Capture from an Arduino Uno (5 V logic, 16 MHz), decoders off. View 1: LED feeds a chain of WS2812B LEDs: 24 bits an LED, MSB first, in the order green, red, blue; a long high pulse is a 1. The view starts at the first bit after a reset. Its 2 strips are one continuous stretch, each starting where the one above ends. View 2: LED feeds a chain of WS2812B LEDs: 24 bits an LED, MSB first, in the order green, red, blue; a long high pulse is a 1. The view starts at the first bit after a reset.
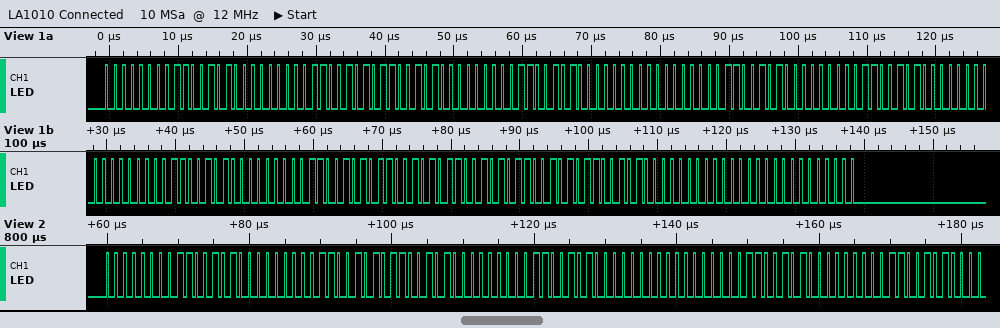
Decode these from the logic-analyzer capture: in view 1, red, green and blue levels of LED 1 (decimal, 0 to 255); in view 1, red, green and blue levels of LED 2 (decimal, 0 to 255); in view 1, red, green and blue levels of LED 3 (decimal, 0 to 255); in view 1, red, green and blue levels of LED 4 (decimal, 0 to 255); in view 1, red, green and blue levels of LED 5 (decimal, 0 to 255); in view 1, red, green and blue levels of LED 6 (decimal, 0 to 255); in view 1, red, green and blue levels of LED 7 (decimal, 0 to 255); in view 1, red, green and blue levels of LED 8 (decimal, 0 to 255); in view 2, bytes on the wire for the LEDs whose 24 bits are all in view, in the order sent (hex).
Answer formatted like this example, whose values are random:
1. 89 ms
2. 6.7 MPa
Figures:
1. 202, 0, 0
2. 202, 202, 0
3. 0, 202, 0
4. 0, 202, 202
5. 0, 0, 202
6. 202, 0, 202
7. 202, 202, 202
8. 0, 0, 0
9. 00 CA 00 CA CA 00 CA 00 00 CA 00 CA
